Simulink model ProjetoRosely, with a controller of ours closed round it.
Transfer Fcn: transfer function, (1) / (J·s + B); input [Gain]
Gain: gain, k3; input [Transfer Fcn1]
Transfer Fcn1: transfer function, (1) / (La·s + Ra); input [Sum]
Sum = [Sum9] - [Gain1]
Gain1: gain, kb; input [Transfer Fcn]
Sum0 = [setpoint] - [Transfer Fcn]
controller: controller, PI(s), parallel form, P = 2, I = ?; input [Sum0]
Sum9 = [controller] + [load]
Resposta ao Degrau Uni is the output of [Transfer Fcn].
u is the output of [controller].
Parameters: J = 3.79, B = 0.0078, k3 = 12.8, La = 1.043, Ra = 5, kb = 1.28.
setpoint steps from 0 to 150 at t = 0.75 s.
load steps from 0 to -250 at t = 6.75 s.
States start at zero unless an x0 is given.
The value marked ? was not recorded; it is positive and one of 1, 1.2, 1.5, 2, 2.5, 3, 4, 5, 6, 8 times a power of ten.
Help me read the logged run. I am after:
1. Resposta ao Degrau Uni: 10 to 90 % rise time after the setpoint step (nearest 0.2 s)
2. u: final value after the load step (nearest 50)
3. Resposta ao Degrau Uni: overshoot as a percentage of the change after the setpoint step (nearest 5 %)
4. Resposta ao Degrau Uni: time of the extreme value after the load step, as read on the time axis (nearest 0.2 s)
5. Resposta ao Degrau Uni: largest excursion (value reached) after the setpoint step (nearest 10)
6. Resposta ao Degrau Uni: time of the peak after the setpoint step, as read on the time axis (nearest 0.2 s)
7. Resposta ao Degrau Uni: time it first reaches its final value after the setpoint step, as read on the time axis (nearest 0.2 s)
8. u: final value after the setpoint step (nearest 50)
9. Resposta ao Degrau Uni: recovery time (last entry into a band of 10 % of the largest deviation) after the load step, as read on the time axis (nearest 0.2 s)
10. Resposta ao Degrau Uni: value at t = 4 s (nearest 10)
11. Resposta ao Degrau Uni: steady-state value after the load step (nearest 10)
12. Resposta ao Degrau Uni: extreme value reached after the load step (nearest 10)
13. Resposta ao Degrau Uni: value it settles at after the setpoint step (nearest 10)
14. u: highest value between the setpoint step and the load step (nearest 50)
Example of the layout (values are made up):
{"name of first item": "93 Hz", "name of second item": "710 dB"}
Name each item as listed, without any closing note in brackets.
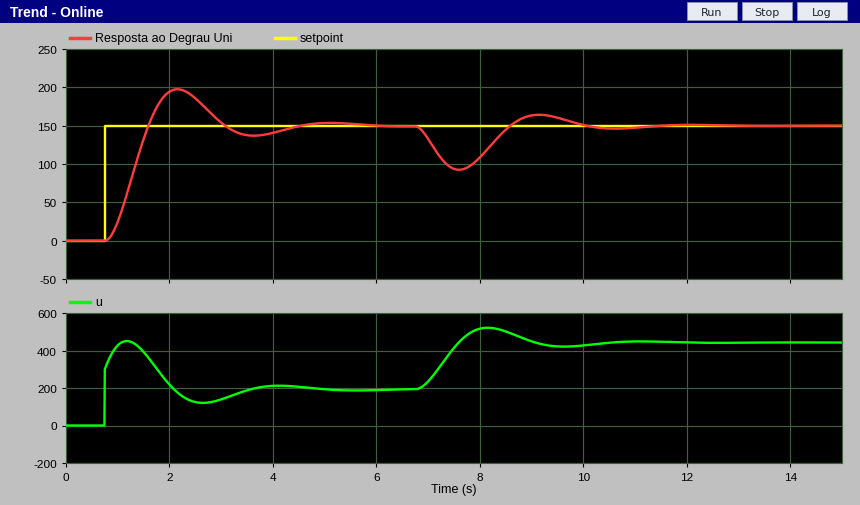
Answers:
{"Resposta ao Degrau Uni: 10 to 90 % rise time after the setpoint step": "0.6 s", "u: final value after the load step": "450", "Resposta ao Degrau Uni: overshoot as a percentage of the change after the setpoint step": "30 %", "Resposta ao Degrau Uni: time of the extreme value after the load step, as read on the time axis": "7.6 s", "Resposta ao Degrau Uni: largest excursion (value reached) after the setpoint step": "200", "Resposta ao Degrau Uni: time of the peak after the setpoint step, as read on the time axis": "2.2 s", "Resposta ao Degrau Uni: time it first reaches its final value after the setpoint step, as read on the time axis": "1.6 s", "u: final value after the setpoint step": "200", "Resposta ao Degrau Uni: recovery time (last entry into a band of 10 % of the largest deviation) after the load step, as read on the time axis": "9.8 s", "Resposta ao Degrau Uni: value at t = 4 s": "140", "Resposta ao Degrau Uni: steady-state value after the load step": "150", "Resposta ao Degrau Uni: extreme value reached after the load step": "90", "Resposta ao Degrau Uni: value it settles at after the setpoint step": "150", "u: highest value between the setpoint step and the load step": "450"}
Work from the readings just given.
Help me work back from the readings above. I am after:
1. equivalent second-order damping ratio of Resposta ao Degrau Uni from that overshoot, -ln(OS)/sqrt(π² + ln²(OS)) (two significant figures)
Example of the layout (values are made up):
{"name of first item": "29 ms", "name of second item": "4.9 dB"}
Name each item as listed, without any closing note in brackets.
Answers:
{"equivalent second-order damping ratio of Resposta ao Degrau Uni from that overshoot, -ln(OS)/sqrt(π² + ln²(OS))": "0.36"}
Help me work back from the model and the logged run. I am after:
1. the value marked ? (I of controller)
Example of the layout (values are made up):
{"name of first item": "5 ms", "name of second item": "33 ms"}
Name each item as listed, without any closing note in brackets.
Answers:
{"the value marked ?": "5"}
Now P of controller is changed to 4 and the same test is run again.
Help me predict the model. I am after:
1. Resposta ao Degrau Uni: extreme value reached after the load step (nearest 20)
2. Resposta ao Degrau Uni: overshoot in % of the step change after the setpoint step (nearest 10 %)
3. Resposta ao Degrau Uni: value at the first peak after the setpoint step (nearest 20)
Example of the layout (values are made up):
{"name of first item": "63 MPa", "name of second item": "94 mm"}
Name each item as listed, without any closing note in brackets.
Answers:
{"Resposta ao Degrau Uni: extreme value reached after the load step": "100", "Resposta ao Degrau Uni: overshoot in % of the step change after the setpoint step": "20 %", "Resposta ao Degrau Uni: value at the first peak after the setpoint step": "180"}
